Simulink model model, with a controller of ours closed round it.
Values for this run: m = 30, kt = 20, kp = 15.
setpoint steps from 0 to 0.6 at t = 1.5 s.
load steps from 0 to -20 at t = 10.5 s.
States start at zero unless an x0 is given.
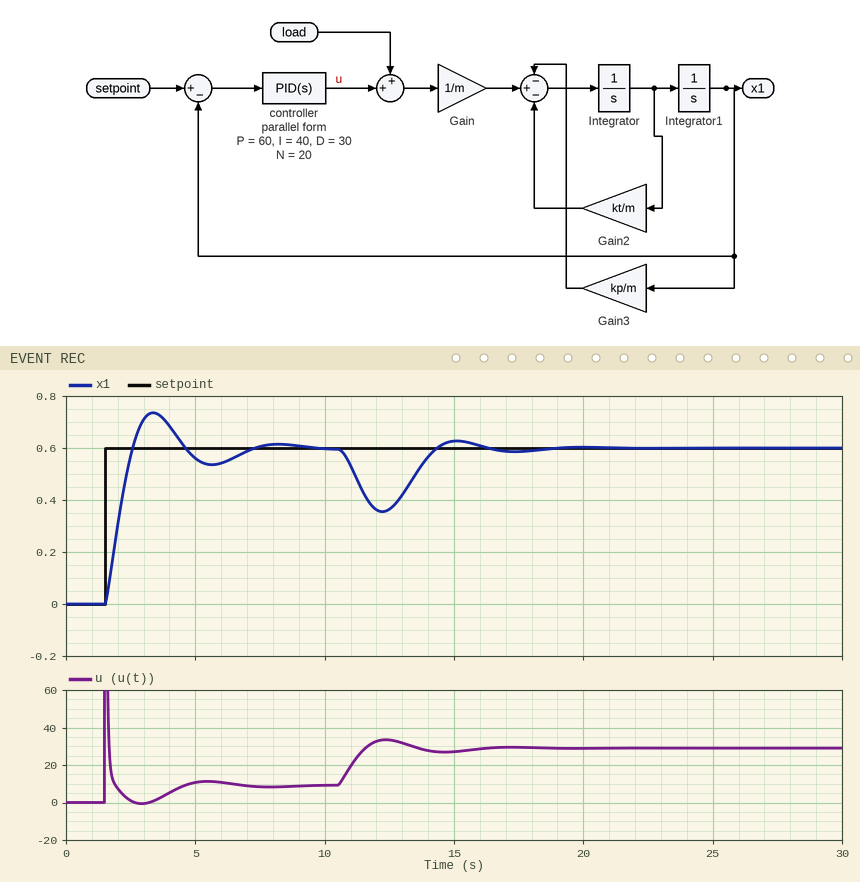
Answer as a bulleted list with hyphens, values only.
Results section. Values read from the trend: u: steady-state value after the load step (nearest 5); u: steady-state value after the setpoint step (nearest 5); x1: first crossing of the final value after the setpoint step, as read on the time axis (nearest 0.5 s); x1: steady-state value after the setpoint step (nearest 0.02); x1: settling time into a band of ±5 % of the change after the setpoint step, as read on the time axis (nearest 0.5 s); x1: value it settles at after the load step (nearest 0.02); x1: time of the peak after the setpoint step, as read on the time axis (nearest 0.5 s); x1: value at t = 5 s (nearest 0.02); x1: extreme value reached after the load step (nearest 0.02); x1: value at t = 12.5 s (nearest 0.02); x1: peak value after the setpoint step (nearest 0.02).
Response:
- 30
- 10
- 2.5 s
- 0.60
- 6.5 s
- 0.60
- 3.5 s
- 0.56
- 0.36
- 0.36
- 0.74
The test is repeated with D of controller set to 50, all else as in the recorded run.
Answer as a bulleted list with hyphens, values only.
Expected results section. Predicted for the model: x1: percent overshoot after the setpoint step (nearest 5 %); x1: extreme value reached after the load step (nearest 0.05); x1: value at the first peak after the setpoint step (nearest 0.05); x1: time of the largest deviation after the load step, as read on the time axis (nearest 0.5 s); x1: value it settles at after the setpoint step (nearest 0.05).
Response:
- 10 %
- 0.40
- 0.65
- 12.5 s
- 0.60
